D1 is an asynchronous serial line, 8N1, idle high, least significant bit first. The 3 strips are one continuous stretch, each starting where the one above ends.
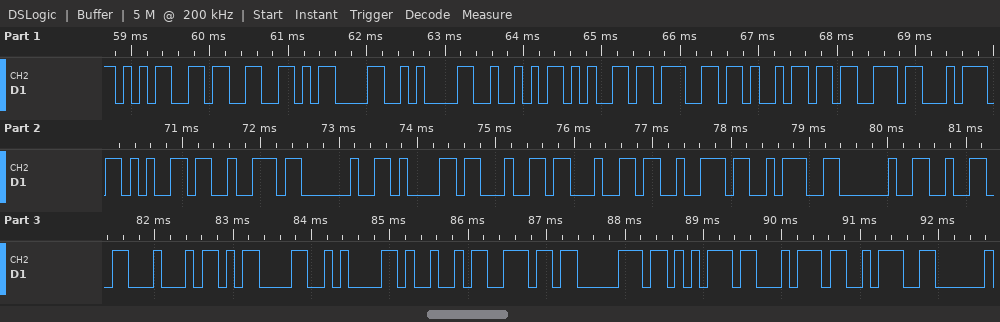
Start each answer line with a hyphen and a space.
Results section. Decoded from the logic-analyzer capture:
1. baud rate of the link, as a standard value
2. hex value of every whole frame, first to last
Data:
- 9600 baud
- 35 33 0D 0A 52 65 67 69 73 74 65 72 20 61 64 64 72 3A 20 32 44 0D 0A 49 6E 70 75 74 3A
